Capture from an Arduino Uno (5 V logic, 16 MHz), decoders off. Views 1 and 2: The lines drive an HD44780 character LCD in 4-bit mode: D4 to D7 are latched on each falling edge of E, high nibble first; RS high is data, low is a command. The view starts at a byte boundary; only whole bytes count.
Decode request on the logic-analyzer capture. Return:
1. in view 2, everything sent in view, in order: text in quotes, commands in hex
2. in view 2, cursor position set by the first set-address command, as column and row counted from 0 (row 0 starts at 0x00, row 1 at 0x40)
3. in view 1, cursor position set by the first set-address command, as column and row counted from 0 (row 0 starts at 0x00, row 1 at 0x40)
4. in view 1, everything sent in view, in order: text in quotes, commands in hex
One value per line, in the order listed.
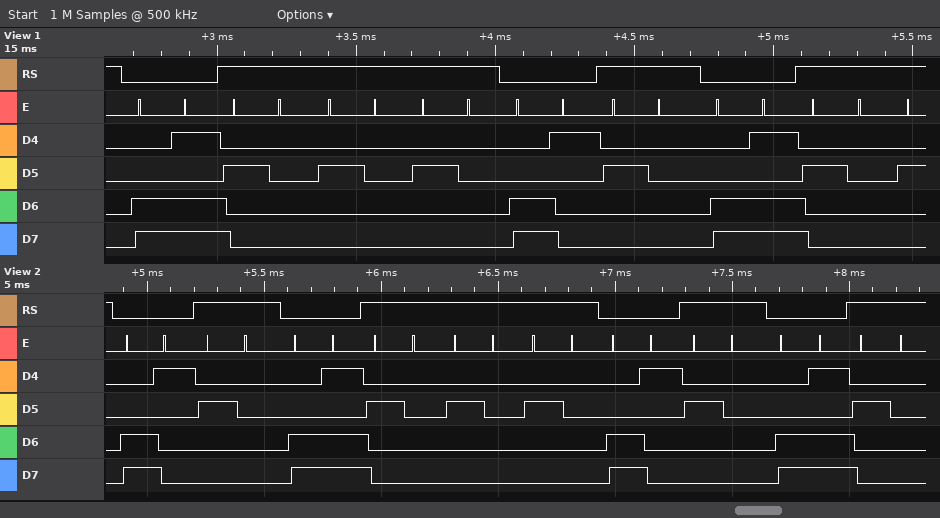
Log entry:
0xC1 " " 0xCD "   " 0xC1 " " 0xCD " "
column 1, row 1
column 13, row 1
0xCD "   " 0xC1 " " 0xCD " "
